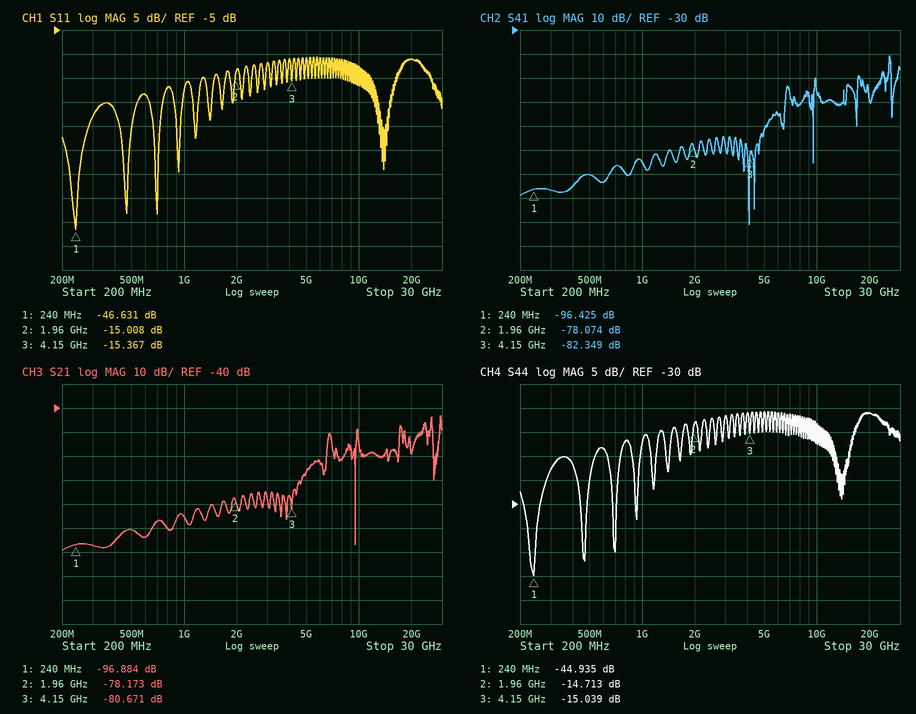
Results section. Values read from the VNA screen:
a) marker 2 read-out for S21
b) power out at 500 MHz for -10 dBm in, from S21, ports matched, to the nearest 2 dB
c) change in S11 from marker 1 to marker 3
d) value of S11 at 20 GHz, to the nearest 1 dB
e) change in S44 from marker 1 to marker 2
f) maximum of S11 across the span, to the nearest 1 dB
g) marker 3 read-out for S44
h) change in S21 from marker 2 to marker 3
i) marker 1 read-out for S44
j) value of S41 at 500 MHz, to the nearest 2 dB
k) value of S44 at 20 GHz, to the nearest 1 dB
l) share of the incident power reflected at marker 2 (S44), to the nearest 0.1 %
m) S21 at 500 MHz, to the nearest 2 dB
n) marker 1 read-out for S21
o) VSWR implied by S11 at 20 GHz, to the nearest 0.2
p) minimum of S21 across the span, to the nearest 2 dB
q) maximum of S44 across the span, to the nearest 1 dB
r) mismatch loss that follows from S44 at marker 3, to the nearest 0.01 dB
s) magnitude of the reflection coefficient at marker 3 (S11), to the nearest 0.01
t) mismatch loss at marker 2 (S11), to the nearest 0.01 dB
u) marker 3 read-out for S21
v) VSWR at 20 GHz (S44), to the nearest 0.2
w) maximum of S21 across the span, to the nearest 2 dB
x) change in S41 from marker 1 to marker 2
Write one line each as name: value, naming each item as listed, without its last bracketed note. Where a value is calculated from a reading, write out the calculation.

marker 2 read-out for S21: -78.173 dB
power out at 500 MHz for -10 dBm in, from S21, ports matched, to the nearest 2 dB: -10 dBm + (-90 dB) = -100 dBm
change in S11 from marker 1 to marker 3: -15.367 − (-46.631) = 31.264 dB
value of S11 at 20 GHz, to the nearest 1 dB: -11 dB
change in S44 from marker 1 to marker 2: -14.713 − (-44.935) = 30.222 dB
maximum of S11 across the span, to the nearest 1 dB: -11 dB
marker 3 read-out for S44: -15.039 dB
change in S21 from marker 2 to marker 3: -80.671 − (-78.173) = -2.498 dB
marker 1 read-out for S44: -44.935 dB
value of S41 at 500 MHz, to the nearest 2 dB: -90 dB
value of S44 at 20 GHz, to the nearest 1 dB: -11 dB
share of the incident power reflected at marker 2 (S44), to the nearest 0.1 %: 10^(-14.713/10) ≈ 3.4 %
S21 at 500 MHz, to the nearest 2 dB: -90 dB
marker 1 read-out for S21: -96.884 dB
VSWR implied by S11 at 20 GHz, to the nearest 0.2: |Γ| = 10^(-11/20) = 0.2818; VSWR = (1 + 0.2818)/(1 − 0.2818) ≈ 1.8
minimum of S21 across the span, to the nearest 2 dB: -100 dB
maximum of S44 across the span, to the nearest 1 dB: -11 dB
mismatch loss that follows from S44 at marker 3, to the nearest 0.01 dB: −10 log10(1 − 10^(-15.039/10)) ≈ 0.14 dB
magnitude of the reflection coefficient at marker 3 (S11), to the nearest 0.01: 10^(-15.367/20) ≈ 0.17
mismatch loss at marker 2 (S11), to the nearest 0.01 dB: −10 log10(1 − 10^(-15.008/10)) ≈ 0.14 dB
marker 3 read-out for S21: -80.671 dB
VSWR at 20 GHz (S44), to the nearest 0.2: |Γ| = 10^(-11/20) = 0.2818; VSWR = (1 + 0.2818)/(1 − 0.2818) ≈ 1.8
maximum of S21 across the span, to the nearest 2 dB: -44 dB
change in S41 from marker 1 to marker 2: -78.074 − (-96.425) = 18.351 dB
